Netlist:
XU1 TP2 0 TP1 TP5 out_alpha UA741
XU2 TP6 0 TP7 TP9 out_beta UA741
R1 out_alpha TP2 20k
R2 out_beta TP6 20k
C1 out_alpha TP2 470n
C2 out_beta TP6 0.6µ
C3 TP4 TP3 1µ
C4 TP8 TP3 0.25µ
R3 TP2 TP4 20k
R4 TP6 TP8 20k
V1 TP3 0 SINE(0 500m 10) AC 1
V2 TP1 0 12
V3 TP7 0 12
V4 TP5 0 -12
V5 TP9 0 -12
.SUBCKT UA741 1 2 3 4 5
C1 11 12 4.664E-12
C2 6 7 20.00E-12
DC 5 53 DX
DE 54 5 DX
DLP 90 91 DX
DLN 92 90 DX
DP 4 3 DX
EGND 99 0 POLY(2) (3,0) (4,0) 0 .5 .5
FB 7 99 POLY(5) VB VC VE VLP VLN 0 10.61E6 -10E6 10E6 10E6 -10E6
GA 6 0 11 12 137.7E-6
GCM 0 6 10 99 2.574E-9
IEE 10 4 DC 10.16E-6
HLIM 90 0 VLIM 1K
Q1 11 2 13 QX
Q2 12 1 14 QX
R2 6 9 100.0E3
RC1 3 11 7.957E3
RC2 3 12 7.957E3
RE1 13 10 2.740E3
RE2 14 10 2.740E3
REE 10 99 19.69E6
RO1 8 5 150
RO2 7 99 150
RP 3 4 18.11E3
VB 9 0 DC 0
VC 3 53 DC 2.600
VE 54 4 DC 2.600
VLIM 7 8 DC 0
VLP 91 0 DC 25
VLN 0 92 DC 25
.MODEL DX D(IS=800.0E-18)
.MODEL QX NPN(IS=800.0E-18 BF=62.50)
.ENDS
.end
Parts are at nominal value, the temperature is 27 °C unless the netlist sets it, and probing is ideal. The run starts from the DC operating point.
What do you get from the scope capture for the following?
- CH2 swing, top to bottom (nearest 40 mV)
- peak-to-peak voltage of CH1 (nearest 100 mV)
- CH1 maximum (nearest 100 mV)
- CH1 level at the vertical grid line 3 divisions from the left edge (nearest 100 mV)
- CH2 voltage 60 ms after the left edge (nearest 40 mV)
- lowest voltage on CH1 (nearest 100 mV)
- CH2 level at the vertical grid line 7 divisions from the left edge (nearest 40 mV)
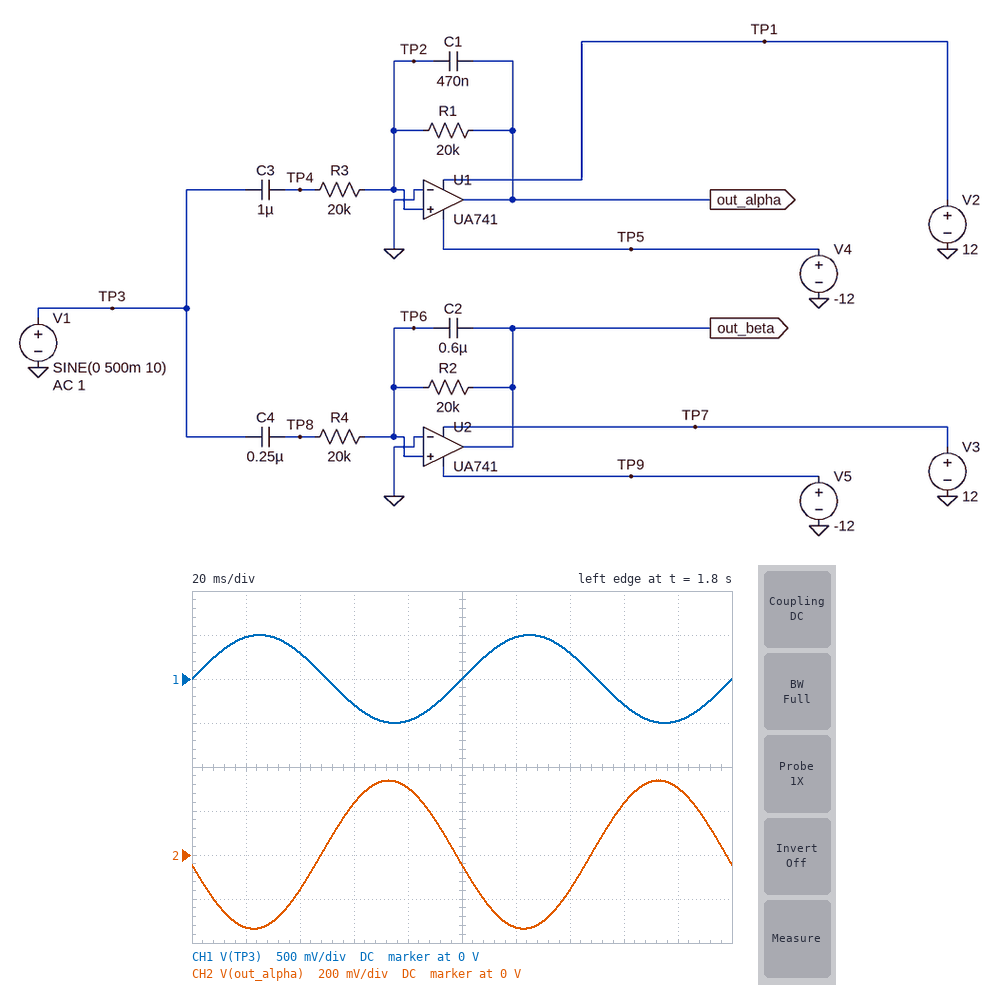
680 mV
1.0 V
500 mV
-300 mV
240 mV
-500 mV
-160 mV
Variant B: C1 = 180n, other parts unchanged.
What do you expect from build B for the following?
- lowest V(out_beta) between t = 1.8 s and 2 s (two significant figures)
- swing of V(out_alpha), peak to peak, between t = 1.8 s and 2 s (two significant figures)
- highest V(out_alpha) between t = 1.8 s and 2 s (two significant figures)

-120 mV
760 mV
380 mV
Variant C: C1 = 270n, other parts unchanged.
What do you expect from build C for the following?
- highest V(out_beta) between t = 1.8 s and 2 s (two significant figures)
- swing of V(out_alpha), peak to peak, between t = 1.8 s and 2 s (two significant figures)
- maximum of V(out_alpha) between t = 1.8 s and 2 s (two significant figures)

120 mV
740 mV
370 mV
